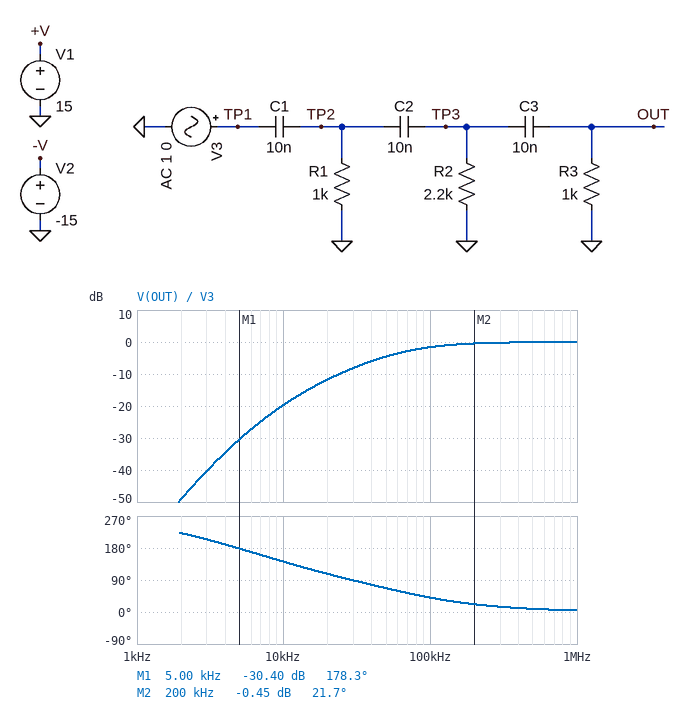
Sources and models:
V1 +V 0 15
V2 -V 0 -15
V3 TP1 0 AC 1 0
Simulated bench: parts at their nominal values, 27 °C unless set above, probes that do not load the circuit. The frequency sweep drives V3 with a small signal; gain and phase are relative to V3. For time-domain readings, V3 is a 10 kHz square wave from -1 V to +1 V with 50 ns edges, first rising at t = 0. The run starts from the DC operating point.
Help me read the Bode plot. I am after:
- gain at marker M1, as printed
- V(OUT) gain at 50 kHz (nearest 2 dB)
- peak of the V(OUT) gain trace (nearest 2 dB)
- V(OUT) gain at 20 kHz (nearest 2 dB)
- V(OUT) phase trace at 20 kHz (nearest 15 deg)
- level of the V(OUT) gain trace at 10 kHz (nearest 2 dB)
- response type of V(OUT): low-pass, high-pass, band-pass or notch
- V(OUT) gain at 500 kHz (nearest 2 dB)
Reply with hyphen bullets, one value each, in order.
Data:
- -30.40 dB
- -4 dB
- 0 dB
- -12 dB
- 105 deg
- -20 dB
- high-pass
- 0 dB
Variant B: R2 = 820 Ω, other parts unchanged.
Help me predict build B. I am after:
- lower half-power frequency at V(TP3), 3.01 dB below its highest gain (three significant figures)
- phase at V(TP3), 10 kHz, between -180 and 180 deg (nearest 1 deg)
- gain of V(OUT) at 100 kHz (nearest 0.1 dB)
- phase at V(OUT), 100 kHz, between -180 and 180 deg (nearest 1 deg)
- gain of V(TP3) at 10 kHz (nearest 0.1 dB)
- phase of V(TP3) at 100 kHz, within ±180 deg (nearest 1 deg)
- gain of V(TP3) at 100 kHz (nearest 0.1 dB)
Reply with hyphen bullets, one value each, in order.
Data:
- 85.3 kHz
- 100 deg
- -2.5 dB
- 50 deg
- -17.7 dB
- 41 deg
- -2.4 dB
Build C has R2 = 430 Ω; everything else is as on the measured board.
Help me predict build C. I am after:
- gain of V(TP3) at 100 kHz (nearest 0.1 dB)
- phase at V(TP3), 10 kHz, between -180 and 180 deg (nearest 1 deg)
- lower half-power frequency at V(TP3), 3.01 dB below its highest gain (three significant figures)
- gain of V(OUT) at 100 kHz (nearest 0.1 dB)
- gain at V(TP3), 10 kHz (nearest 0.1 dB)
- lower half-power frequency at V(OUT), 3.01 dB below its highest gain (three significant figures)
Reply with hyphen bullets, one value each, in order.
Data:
- -3.8 dB
- 111 deg
- 119 kHz
- -3.9 dB
- -21.4 dB
- 121 kHz
